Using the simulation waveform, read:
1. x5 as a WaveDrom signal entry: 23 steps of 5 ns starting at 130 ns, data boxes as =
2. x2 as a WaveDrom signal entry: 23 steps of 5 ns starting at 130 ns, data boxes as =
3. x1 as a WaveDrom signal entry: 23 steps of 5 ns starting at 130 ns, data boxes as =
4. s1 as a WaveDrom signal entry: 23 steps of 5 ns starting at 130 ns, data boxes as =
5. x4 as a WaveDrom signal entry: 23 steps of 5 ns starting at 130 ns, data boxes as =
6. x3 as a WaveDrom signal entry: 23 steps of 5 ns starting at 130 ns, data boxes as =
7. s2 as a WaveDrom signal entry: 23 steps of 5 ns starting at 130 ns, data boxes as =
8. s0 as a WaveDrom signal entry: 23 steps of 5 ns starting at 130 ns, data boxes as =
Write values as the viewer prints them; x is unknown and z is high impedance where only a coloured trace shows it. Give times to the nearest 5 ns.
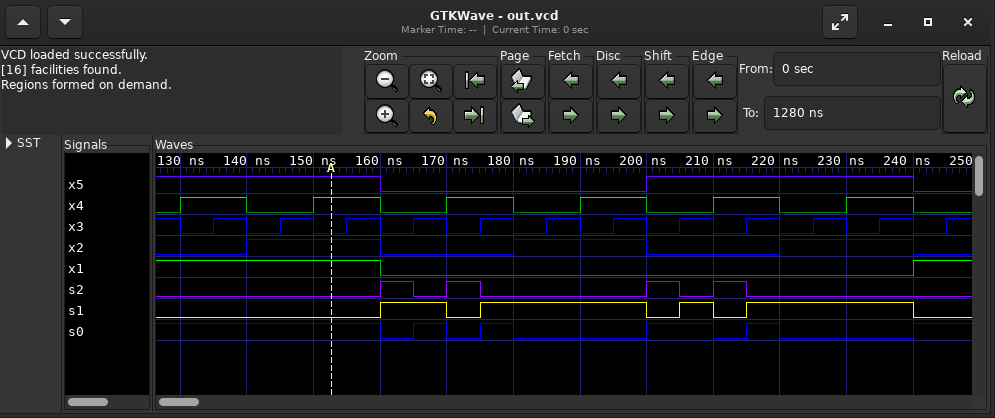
{name: 'x5', wave: '1.....0.......1.......0'}
{name: 'x2', wave: '0.1...0...1...0...1...0'}
{name: 'x1', wave: '1.....0...............1'}
{name: 's1', wave: '0.....1.01....0101....0'}
{name: 'x4', wave: '1.0.1.0.1.0.1.0.1.0.1.0'}
{name: 'x3', wave: '01010101010101010101010'}
{name: 's2', wave: '0.....1010....1010.....'}
{name: 's0', wave: '1.....01010...1.010...1'}
